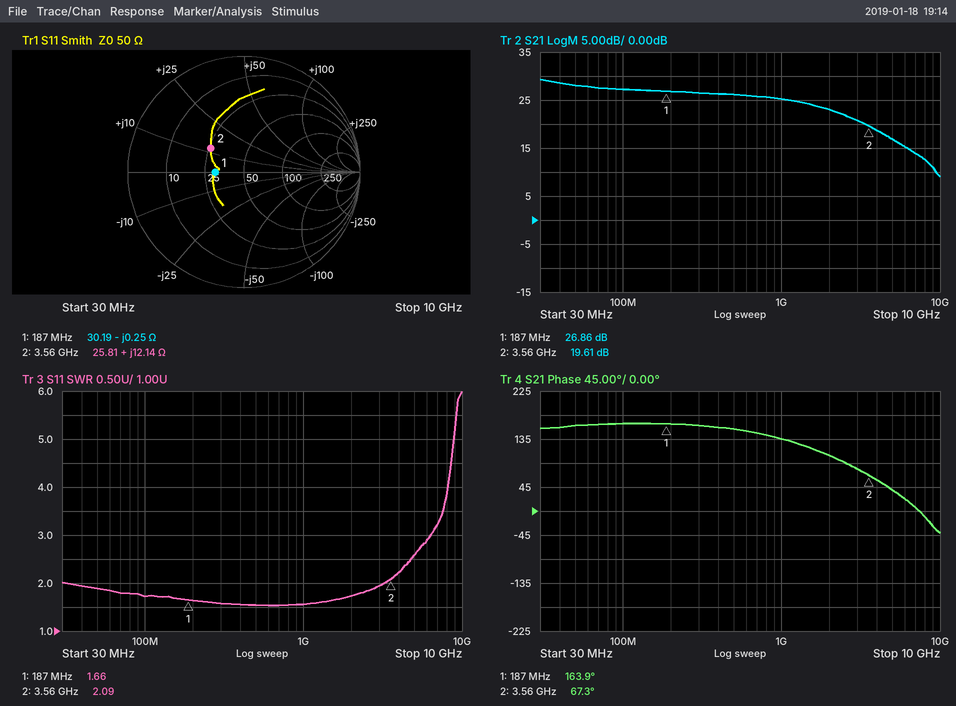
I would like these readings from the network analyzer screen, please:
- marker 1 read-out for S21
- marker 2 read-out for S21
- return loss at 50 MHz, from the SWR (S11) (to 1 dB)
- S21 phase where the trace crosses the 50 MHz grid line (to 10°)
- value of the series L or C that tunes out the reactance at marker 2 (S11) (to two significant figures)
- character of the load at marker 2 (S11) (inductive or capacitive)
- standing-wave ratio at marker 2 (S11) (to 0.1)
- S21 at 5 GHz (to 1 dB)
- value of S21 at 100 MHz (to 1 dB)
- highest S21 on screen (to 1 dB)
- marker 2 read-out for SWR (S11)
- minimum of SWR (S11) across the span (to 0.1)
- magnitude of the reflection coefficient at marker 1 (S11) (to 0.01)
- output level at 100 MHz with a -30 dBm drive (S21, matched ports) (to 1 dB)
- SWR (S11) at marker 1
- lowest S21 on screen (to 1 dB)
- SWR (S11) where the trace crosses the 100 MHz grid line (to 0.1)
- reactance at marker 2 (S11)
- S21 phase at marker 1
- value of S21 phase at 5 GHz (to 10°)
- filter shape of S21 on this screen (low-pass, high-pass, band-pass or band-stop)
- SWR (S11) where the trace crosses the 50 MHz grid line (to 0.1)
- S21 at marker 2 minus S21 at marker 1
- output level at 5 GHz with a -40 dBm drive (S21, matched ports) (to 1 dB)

26.86 dB
19.61 dB
10 dB
160°
3.7 pF
inductive
2.1
17 dB
27 dB
29 dB
2.09
1.5
0.25
-3 dBm
1.66
9 dB
1.7
+12.14 Ω
163.9°
40°
low-pass
1.9
-7.25 dB
-23 dBm
